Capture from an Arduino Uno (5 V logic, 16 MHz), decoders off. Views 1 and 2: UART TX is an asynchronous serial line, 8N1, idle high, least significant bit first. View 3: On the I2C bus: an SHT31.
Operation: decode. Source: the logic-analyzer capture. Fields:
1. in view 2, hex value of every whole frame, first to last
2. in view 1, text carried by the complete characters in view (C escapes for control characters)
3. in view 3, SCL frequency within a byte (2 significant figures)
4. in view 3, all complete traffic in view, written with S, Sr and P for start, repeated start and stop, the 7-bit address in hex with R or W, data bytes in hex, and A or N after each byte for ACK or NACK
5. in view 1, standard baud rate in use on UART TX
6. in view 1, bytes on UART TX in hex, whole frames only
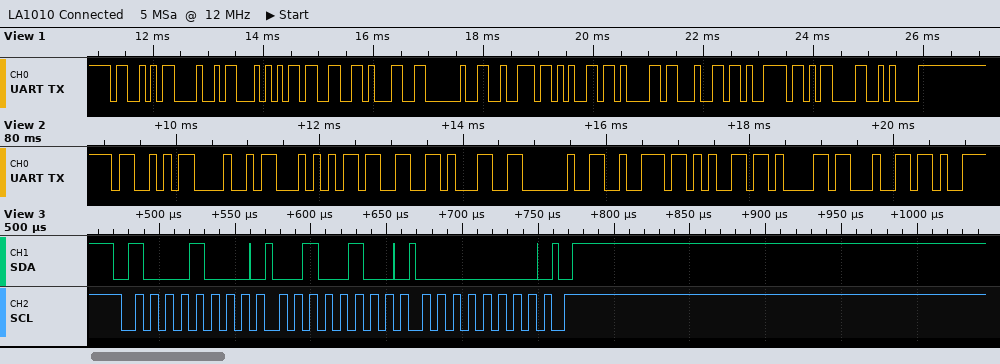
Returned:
0x53 0x48 0x54 0x33 0x31 0x20 0x72 0x65 0x61 0x64
"SHT31 ready\r\n"
100 kHz
S 44W A 24 A 00 A P
9600 baud
53 48 54 33 31 20 72 65 61 64 79 0D 0A
